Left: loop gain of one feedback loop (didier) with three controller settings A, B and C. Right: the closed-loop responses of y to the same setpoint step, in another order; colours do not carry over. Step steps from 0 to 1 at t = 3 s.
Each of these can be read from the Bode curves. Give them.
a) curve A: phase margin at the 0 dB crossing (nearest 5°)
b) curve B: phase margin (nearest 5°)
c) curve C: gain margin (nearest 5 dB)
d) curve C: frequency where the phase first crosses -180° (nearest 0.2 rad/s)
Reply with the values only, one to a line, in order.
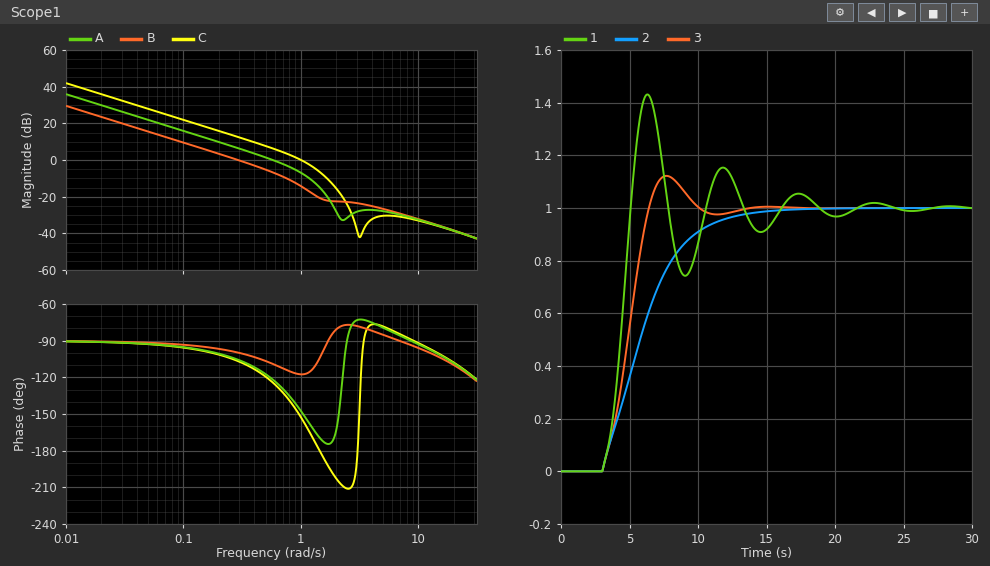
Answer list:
60°
80°
5 dB
1.4 rad/s
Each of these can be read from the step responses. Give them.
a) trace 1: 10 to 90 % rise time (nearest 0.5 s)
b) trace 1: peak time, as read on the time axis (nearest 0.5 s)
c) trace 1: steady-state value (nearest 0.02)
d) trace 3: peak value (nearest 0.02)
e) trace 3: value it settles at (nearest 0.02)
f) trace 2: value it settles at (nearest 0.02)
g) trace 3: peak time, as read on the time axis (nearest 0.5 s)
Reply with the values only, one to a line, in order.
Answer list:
1.5 s
6.5 s
1.00
1.12
1.00
1.00
7.5 s
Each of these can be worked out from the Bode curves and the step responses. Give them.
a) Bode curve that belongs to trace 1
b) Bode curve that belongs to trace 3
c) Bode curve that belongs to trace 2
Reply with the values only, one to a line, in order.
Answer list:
C
A
B
